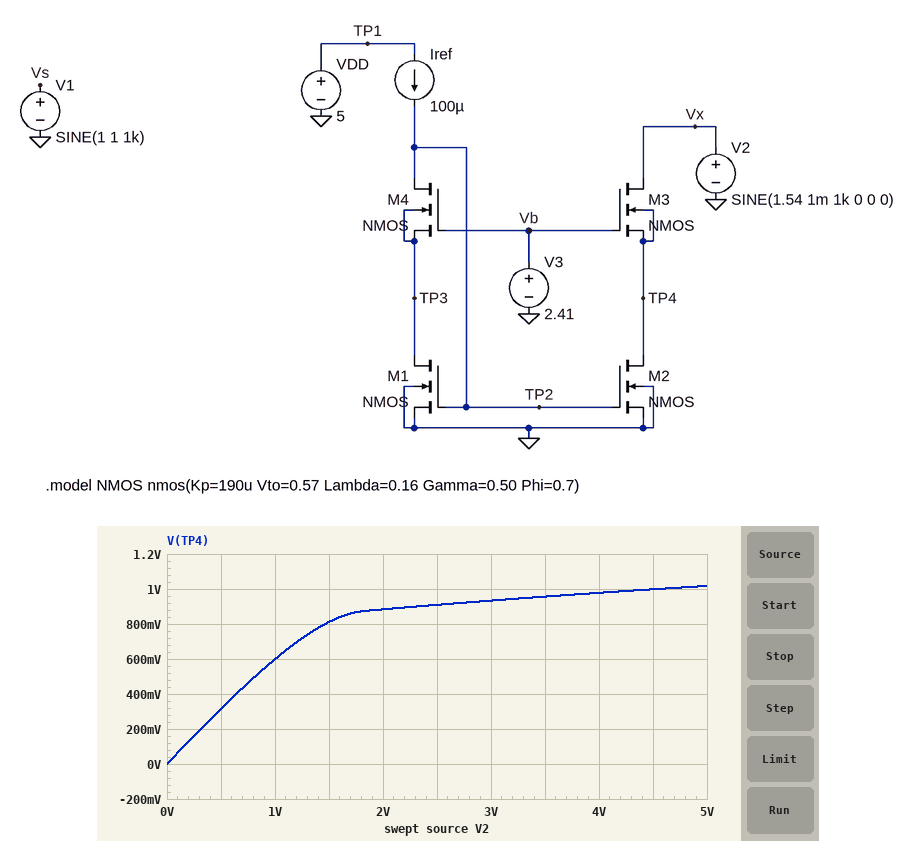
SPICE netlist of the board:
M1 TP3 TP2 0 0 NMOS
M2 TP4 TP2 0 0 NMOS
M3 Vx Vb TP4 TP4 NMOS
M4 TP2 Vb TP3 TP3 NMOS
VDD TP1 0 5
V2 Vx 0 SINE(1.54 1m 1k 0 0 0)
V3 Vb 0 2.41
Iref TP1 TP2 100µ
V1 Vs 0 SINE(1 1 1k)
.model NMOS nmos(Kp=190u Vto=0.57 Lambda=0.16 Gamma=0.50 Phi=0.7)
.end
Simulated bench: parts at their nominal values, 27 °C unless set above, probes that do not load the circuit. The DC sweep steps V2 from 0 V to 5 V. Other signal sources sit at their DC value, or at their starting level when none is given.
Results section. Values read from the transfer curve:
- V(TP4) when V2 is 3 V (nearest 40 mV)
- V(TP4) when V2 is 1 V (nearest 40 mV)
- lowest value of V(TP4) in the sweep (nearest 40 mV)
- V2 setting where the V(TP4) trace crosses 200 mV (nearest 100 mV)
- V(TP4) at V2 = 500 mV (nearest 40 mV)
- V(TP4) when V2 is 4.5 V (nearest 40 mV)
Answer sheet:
920 mV
600 mV
0 V
300 mV
320 mV
1.00 V
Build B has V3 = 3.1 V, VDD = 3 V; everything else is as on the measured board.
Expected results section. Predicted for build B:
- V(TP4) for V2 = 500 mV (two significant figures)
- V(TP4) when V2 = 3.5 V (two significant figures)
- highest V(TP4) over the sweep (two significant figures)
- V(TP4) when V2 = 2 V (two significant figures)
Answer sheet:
360 mV
1.6 V
1.7 V
1.4 V
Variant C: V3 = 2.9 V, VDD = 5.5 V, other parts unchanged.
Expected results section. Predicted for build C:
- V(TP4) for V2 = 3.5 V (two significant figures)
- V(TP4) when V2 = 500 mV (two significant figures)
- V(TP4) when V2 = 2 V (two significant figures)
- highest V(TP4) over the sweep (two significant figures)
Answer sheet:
1.4 V
350 mV
1.3 V
1.5 V
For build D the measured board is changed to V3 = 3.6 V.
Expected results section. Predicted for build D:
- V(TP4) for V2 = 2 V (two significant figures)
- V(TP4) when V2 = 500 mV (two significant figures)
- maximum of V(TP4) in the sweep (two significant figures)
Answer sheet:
1.6 V
380 mV
2.1 V
